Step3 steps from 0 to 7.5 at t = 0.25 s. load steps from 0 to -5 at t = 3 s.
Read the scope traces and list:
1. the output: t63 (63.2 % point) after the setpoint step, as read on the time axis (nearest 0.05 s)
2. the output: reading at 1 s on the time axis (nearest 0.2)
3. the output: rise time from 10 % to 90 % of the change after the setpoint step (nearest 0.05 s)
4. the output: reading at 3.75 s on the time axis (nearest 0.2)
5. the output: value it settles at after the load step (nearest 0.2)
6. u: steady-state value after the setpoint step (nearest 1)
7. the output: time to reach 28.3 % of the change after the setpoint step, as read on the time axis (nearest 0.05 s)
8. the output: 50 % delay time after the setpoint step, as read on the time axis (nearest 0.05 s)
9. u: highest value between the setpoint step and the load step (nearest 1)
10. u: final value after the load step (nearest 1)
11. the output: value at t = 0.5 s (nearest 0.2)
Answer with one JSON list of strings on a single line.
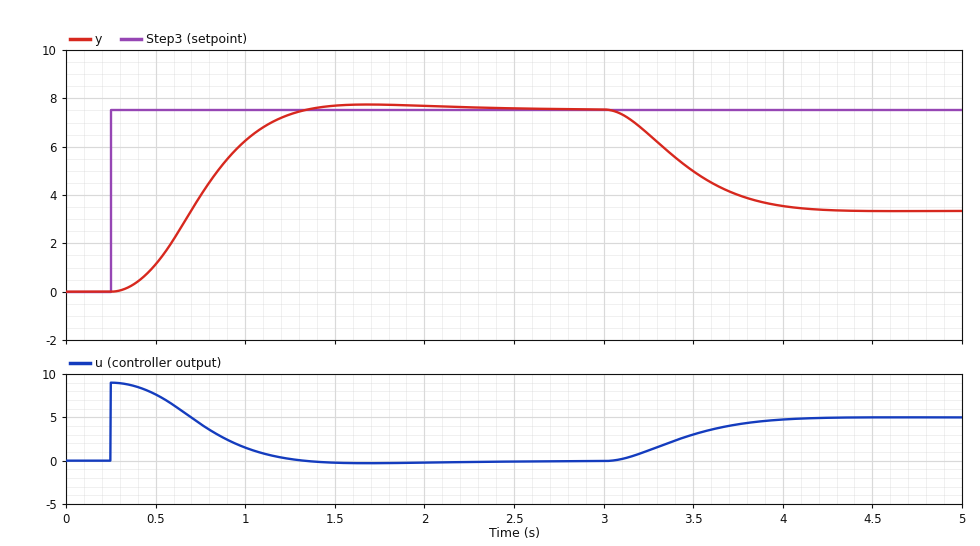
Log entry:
["0.80 s", "6.2", "0.65 s", "4.0", "3.4", "0", "0.60 s", "0.75 s", "9", "5", "1.2"]
